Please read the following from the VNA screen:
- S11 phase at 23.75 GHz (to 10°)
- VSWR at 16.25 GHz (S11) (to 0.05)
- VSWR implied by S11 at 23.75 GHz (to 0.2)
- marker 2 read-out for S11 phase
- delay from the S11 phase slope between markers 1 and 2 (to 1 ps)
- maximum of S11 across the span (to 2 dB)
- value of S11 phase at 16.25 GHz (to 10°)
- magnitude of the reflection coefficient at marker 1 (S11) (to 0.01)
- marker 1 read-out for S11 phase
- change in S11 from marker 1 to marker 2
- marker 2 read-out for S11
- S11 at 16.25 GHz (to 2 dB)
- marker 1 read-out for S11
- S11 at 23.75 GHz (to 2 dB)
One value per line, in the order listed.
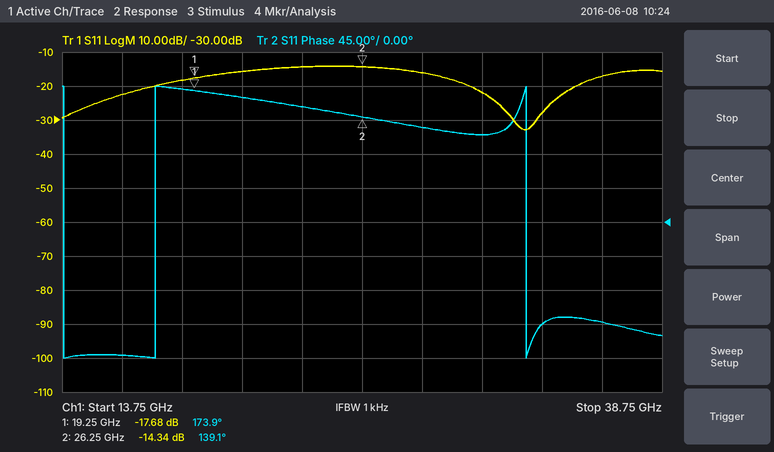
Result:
150°
1.15
1.4
139.1°
14 ps
-14 dB
-180°
0.13
173.9°
3.34 dB
-14.34 dB
-22 dB
-17.68 dB
-14 dB
